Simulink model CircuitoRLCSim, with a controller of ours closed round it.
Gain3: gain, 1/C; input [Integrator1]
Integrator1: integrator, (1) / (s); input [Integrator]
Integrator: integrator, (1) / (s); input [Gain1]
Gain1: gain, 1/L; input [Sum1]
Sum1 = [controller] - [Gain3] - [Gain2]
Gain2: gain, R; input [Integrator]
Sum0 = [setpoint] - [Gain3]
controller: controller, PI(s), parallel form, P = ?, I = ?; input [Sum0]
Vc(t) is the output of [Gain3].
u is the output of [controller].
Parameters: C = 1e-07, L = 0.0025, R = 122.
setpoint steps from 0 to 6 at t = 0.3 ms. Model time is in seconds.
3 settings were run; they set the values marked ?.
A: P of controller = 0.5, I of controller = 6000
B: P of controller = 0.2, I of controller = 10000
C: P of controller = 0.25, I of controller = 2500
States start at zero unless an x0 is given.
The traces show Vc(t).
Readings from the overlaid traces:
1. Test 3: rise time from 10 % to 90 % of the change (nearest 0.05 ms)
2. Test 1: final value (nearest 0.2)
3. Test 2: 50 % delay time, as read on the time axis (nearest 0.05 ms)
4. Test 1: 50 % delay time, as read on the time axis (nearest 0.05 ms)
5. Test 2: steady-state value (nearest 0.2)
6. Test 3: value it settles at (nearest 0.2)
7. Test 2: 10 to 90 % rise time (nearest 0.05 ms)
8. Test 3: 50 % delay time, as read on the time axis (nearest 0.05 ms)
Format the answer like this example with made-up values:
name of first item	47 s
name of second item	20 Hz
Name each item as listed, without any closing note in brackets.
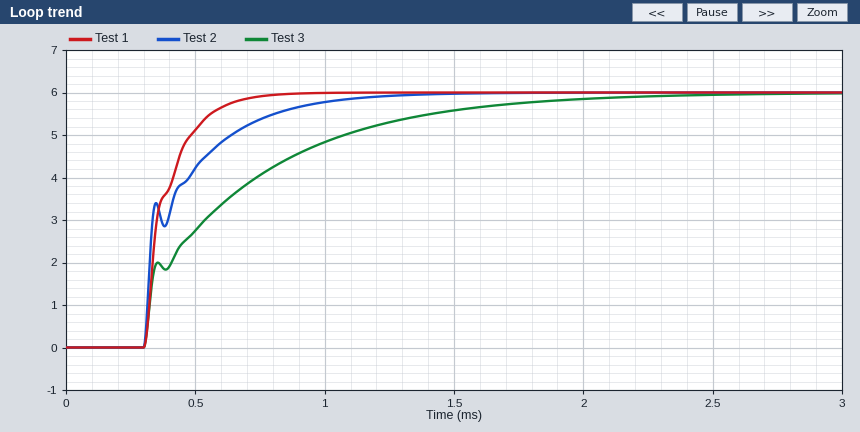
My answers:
Test 3: rise time from 10 % to 90 % of the change	1.00 ms
Test 1: final value	6.0
Test 2: 50 % delay time, as read on the time axis	0.35 ms
Test 1: 50 % delay time, as read on the time axis	0.35 ms
Test 2: steady-state value	6.0
Test 3: value it settles at	6.0
Test 2: 10 to 90 % rise time	0.45 ms
Test 3: 50 % delay time, as read on the time axis	0.55 ms
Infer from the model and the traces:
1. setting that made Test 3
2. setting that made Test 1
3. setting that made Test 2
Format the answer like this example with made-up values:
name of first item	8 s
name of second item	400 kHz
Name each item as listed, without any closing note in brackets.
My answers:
setting that made Test 3	C
setting that made Test 1	B
setting that made Test 2	A
